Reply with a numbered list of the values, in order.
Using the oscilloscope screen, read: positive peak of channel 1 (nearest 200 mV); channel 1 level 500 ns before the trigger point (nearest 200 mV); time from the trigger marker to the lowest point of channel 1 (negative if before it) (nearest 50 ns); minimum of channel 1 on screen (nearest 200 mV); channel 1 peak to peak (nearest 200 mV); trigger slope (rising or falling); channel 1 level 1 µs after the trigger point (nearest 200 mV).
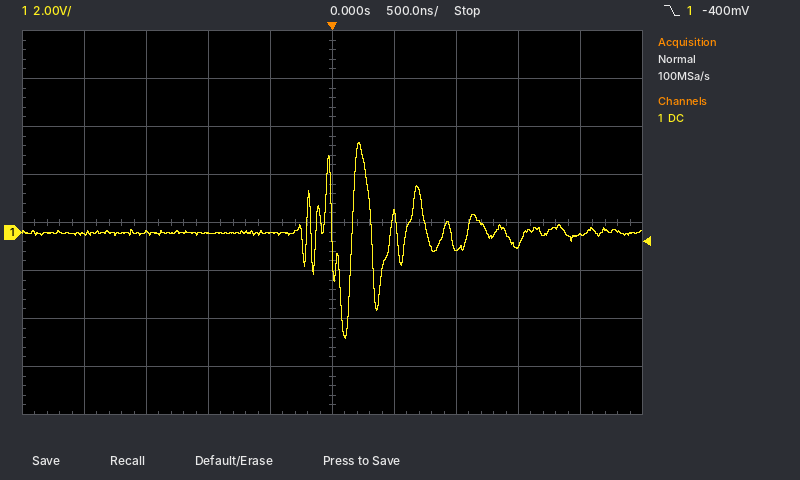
1. 3.8 V
2. 0.0 V
3. +100 ns
4. -4.4 V
5. 8.2 V
6. falling
7. -600 mV
